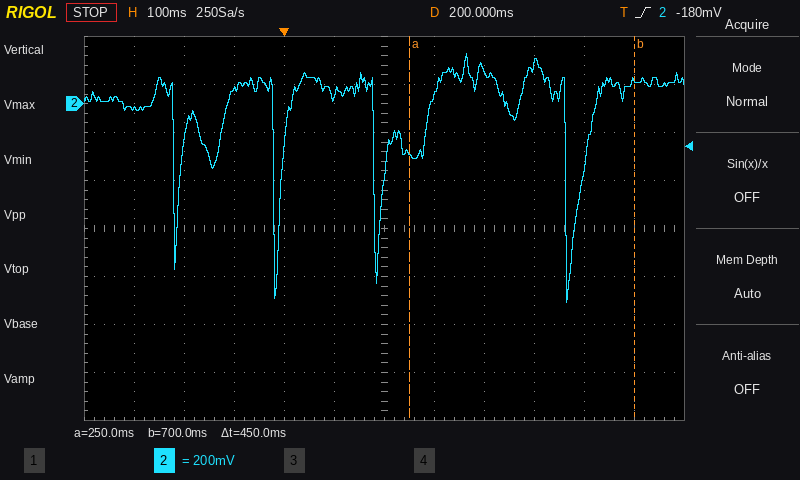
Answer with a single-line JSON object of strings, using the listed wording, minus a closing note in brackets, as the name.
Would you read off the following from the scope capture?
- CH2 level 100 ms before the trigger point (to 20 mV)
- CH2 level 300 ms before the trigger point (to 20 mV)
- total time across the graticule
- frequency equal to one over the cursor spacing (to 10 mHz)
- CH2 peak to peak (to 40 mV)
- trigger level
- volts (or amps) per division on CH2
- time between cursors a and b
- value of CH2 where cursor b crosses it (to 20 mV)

{"CH2 level 100 ms before the trigger point": "60 mV", "CH2 level 300 ms before the trigger point": "-20 mV", "total time across the graticule": "1.2 s", "frequency equal to one over the cursor spacing": "2.22 Hz", "CH2 peak to peak": "1.04 V", "trigger level": "-180 mV", "volts (or amps) per division on CH2": "200 mV", "time between cursors a and b": "450 ms", "value of CH2 where cursor b crosses it": "100 mV"}
